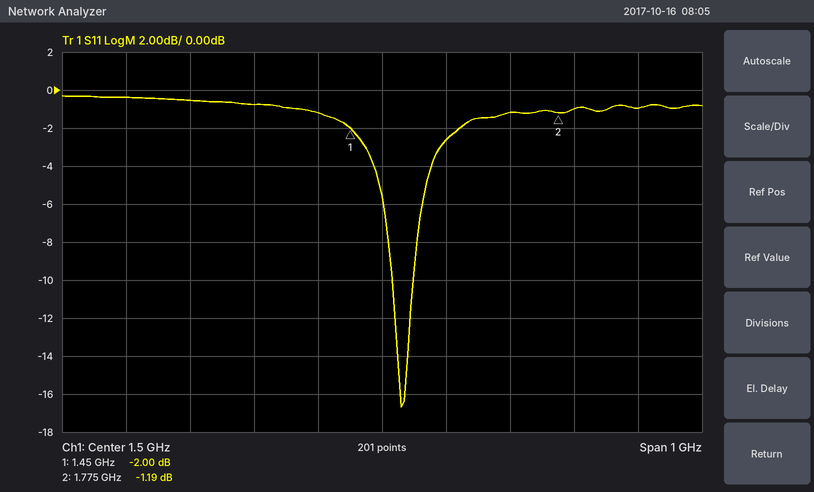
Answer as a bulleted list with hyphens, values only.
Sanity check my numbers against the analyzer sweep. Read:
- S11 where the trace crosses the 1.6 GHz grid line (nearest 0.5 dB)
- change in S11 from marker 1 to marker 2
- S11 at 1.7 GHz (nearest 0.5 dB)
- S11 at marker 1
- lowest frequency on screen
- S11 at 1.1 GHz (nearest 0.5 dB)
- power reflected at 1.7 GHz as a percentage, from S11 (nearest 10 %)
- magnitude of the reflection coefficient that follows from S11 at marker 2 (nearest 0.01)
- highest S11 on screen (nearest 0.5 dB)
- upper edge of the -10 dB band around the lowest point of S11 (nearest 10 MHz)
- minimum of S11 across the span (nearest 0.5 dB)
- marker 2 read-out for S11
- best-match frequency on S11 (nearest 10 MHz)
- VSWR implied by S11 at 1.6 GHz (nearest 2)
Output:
- -2.5 dB
- 0.81 dB
- -1.0 dB
- -2.00 dB
- 1 GHz
- -0.5 dB
- 80 %
- 0.87
- -0.5 dB
- 1.55 GHz
- -16.5 dB
- -1.19 dB
- 1.53 GHz
- 6
